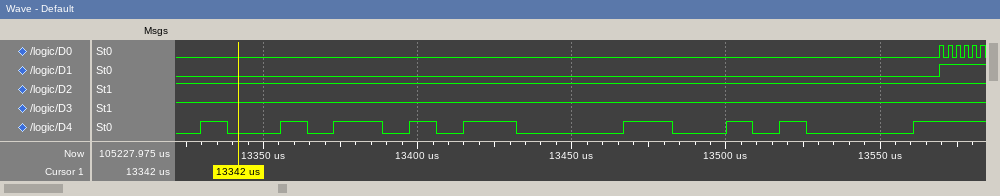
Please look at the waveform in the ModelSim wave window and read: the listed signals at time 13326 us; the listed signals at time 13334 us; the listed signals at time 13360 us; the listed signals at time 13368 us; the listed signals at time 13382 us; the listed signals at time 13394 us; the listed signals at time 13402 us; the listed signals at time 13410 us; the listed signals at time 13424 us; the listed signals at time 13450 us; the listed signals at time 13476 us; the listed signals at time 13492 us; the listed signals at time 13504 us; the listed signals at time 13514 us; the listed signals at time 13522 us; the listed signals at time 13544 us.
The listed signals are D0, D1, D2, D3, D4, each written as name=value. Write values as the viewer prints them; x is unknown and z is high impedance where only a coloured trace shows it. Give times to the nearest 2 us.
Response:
D0=0, D1=0, D2=1, D3=1, D4=0
D0=0, D1=0, D2=1, D3=1, D4=1
D0=0, D1=0, D2=1, D3=1, D4=1
D0=0, D1=0, D2=1, D3=1, D4=0
D0=0, D1=0, D2=1, D3=1, D4=1
D0=0, D1=0, D2=1, D3=1, D4=0
D0=0, D1=0, D2=1, D3=1, D4=1
D0=0, D1=0, D2=1, D3=1, D4=0
D0=0, D1=0, D2=1, D3=1, D4=1
D0=0, D1=0, D2=1, D3=1, D4=0
D0=0, D1=0, D2=1, D3=1, D4=1
D0=0, D1=0, D2=1, D3=1, D4=0
D0=0, D1=0, D2=1, D3=1, D4=1
D0=0, D1=0, D2=1, D3=1, D4=0
D0=0, D1=0, D2=1, D3=1, D4=1
D0=0, D1=0, D2=1, D3=1, D4=0
